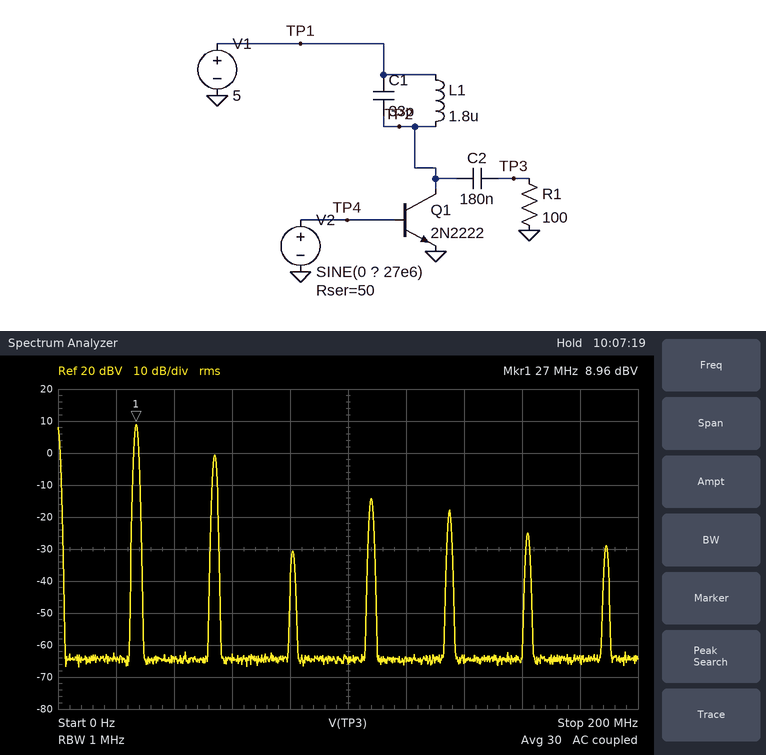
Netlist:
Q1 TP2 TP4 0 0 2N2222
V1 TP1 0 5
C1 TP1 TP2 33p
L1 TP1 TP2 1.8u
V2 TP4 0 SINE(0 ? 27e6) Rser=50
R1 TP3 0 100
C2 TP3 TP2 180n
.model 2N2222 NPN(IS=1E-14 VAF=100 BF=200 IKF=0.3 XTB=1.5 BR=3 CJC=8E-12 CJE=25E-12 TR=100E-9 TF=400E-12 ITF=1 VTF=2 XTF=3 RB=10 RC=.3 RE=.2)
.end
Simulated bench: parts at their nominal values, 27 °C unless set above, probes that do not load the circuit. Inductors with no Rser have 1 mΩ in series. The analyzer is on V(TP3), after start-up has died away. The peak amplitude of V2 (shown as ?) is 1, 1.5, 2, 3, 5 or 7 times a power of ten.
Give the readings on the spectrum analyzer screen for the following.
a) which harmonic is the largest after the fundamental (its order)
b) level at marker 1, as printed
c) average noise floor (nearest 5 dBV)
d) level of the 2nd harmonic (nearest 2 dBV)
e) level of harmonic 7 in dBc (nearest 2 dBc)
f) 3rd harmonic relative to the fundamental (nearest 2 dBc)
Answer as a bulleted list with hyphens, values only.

- 2
- 8.96 dBV
- -65 dBV
- 0 dBV
- -38 dBc
- -40 dBc
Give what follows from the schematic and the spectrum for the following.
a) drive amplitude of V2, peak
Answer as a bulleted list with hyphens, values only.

- 1.5 V
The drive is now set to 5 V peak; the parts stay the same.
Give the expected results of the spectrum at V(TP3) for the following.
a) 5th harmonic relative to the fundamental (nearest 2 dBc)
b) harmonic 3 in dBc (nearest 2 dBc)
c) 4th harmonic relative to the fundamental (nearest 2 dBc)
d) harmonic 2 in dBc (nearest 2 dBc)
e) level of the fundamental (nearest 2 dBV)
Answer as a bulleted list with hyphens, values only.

- -24 dBc
- -26 dBc
- -16 dBc
- -8 dBc
- 14 dBV
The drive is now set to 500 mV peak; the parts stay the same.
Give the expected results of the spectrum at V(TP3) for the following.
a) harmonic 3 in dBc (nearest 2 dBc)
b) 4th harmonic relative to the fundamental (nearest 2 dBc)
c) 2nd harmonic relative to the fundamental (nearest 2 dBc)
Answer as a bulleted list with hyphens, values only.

- -44 dBc
- -58 dBc
- -30 dBc
